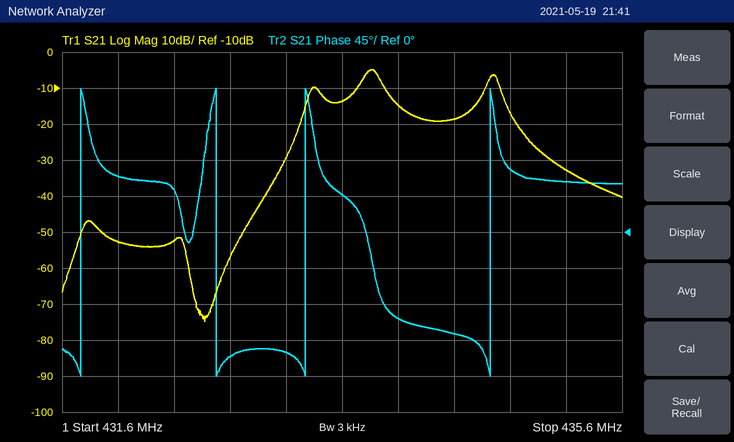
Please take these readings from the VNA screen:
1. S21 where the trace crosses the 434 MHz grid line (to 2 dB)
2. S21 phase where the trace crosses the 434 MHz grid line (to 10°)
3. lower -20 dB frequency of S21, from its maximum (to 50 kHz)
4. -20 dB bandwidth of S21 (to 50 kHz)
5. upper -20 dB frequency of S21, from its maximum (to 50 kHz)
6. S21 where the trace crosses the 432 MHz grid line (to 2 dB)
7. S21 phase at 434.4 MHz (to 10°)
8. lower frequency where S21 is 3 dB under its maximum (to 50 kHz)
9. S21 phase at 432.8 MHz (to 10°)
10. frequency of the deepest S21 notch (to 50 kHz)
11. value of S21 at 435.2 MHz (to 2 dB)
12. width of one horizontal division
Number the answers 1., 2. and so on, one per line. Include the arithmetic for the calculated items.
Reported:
1. -14 dB
2. -110°
3. 433.25 MHz
4. 434.95 MHz − 433.25 MHz = 1.70 MHz
5. 434.95 MHz
6. -52 dB
7. -130°
8. 433.75 MHz
9. -160°
10. 432.60 MHz
11. -32 dB
12. 400 kHz
